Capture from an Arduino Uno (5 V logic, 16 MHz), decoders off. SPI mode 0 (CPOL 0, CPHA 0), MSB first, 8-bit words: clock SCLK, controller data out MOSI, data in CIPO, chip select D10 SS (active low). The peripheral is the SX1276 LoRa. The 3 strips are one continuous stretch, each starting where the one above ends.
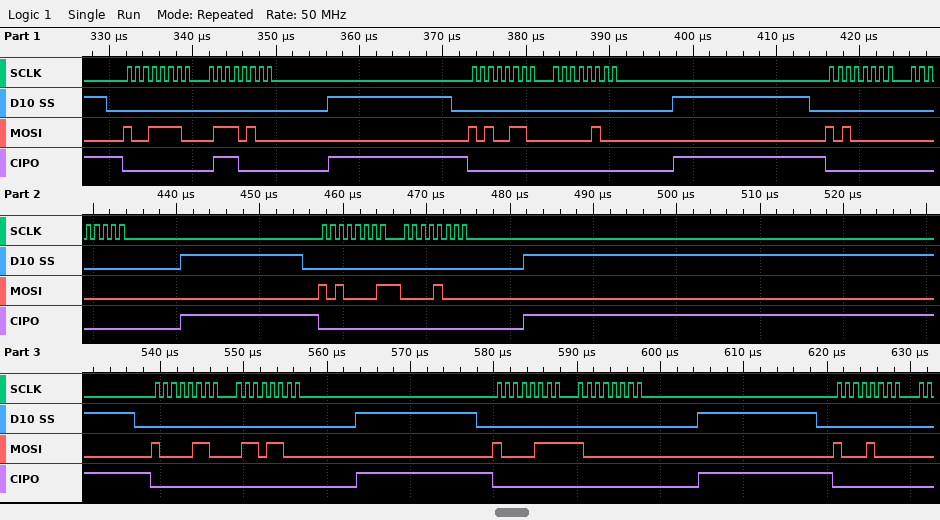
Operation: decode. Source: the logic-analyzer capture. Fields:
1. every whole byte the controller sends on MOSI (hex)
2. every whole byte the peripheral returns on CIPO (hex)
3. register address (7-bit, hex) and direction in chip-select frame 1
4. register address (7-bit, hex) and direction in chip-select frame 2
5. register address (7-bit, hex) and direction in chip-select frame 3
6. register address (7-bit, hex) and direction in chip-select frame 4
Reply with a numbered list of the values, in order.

1. 0x9E 0x74 0xA6 0x04 0xA0 0x00 0xA1 0x08 0x86 0x6C 0x87 0x80 0x88
2. 0x00 0x70 0x00 0x00 0x00 0x00 0x00 0x00 0x00 0x00 0x00 0x00 0x00
3. 0x1E write
4. 0x26 write
5. 0x20 write
6. 0x21 write
